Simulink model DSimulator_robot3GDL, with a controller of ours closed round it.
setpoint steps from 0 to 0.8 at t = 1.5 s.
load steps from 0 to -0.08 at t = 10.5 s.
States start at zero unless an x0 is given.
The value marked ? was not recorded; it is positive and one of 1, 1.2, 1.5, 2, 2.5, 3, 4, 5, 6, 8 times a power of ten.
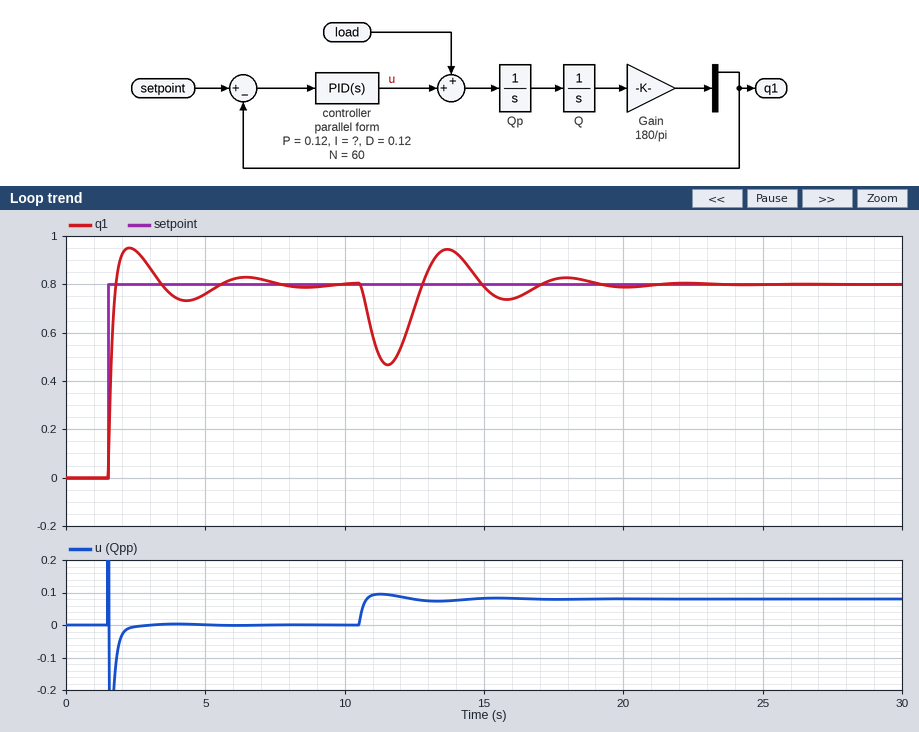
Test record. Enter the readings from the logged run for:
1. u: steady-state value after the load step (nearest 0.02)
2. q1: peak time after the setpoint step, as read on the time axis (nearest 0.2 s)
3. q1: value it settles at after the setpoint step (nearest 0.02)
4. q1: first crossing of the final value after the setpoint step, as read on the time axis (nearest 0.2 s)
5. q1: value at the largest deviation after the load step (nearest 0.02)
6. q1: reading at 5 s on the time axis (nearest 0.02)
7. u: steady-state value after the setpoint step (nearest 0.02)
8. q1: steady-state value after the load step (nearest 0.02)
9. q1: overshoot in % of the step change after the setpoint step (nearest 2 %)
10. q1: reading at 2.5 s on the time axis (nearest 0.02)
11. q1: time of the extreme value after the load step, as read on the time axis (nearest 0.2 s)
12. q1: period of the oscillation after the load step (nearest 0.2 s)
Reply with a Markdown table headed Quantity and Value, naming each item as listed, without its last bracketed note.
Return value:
| Quantity | Value |
|---|---|
| u: steady-state value after the load step | 0.08 |
| q1: peak time after the setpoint step, as read on the time axis | 2.2 s |
| q1: value it settles at after the setpoint step | 0.80 |
| q1: first crossing of the final value after the setpoint step, as read on the time axis | 1.8 s |
| q1: value at the largest deviation after the load step | 0.46 |
| q1: reading at 5 s on the time axis | 0.76 |
| u: steady-state value after the setpoint step | 0.00 |
| q1: steady-state value after the load step | 0.80 |
| q1: overshoot in % of the step change after the setpoint step | 18 % |
| q1: reading at 2.5 s on the time axis | 0.94 |
| q1: time of the extreme value after the load step, as read on the time axis | 11.6 s |
| q1: period of the oscillation after the load step | 4.2 s |
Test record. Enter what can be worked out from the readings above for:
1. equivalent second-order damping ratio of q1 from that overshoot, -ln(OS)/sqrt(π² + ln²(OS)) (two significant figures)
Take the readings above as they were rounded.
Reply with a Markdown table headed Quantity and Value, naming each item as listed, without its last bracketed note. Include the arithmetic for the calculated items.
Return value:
| Quantity | Value |
|---|---|
| equivalent second-order damping ratio of q1 from that overshoot, -ln(OS)/sqrt(π² + ln²(OS)) | ln(0.18) = -1.715; 1.715 / sqrt(9.870 + 2.941) = 0.48 |
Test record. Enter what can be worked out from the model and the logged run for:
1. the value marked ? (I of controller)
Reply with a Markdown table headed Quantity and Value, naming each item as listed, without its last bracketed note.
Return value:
| Quantity | Value |
|---|---|
| the value marked ? | 0.25 |
